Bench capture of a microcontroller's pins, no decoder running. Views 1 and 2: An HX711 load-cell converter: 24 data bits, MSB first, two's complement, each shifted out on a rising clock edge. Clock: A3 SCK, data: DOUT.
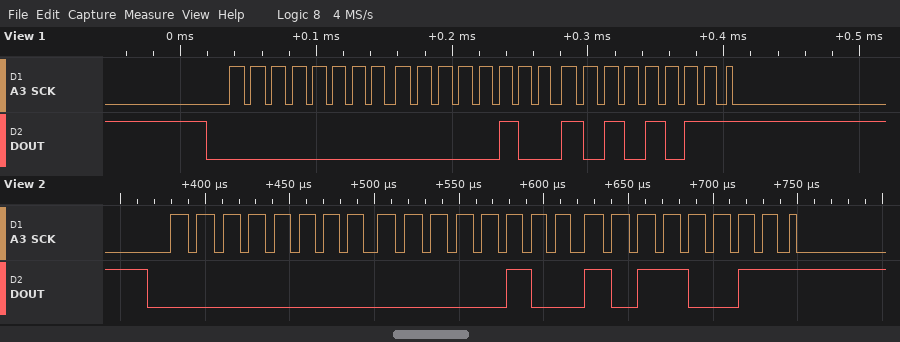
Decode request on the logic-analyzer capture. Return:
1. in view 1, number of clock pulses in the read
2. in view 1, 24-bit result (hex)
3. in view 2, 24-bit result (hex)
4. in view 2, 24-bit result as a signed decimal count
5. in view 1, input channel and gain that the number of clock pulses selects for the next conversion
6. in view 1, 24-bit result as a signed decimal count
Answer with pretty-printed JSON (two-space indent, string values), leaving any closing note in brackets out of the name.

{
  "in view 1, number of clock pulses in the read": "25",
  "in view 1, 24-bit result": "0x0004AB",
  "in view 2, 24-bit result": "0x0004B3",
  "in view 2, 24-bit result as a signed decimal count": "1203",
  "in view 1, input channel and gain that the number of clock pulses selects for the next conversion": "channel A, gain 128",
  "in view 1, 24-bit result as a signed decimal count": "1195"
}
